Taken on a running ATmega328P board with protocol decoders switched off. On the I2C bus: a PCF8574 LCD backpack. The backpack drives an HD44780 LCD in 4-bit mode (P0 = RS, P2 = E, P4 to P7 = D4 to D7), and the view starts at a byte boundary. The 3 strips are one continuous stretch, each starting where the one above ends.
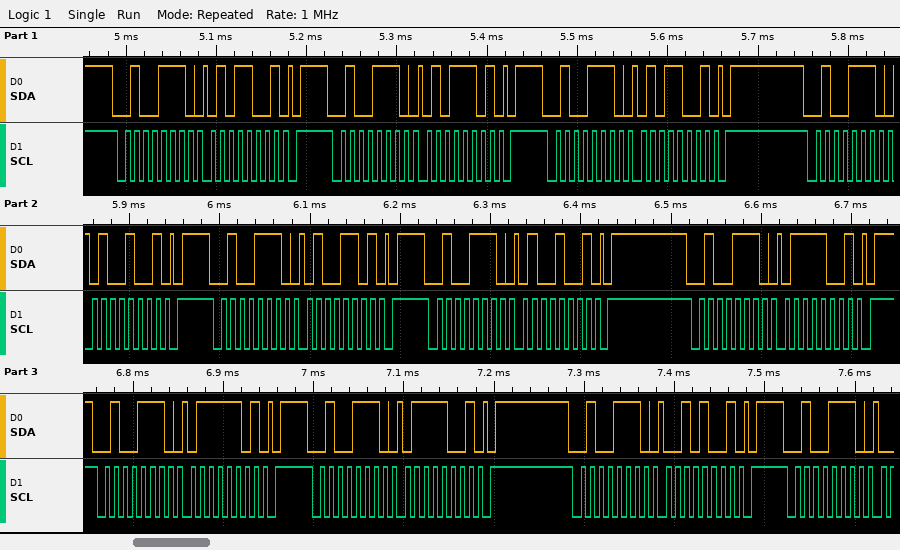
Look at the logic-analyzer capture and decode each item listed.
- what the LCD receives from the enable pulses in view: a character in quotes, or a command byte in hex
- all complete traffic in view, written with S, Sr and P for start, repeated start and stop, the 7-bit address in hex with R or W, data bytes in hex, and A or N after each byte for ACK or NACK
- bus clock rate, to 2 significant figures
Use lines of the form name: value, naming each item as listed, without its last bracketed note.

what the LCD receives from the enable pulses in view: a character in quotes, or a command byte in hex: 'T'
all complete traffic in view, written with S, Sr and P for start, repeated start and stop, the 7-bit address in hex with R or W, data bytes in hex, and A or N after each byte for ACK or NACK: S 27W A 59 A P S 27W A 5D A P S 27W A 59 A P S 27W A 49 A P S 27W A 4D A P S 27W A 49 A P S 27W A 79 A P S 27W A 7D A P S 27W A 79 A P S 27W A 29 A P S 27W A
bus clock rate, to 2 significant figures: 100 kHz
